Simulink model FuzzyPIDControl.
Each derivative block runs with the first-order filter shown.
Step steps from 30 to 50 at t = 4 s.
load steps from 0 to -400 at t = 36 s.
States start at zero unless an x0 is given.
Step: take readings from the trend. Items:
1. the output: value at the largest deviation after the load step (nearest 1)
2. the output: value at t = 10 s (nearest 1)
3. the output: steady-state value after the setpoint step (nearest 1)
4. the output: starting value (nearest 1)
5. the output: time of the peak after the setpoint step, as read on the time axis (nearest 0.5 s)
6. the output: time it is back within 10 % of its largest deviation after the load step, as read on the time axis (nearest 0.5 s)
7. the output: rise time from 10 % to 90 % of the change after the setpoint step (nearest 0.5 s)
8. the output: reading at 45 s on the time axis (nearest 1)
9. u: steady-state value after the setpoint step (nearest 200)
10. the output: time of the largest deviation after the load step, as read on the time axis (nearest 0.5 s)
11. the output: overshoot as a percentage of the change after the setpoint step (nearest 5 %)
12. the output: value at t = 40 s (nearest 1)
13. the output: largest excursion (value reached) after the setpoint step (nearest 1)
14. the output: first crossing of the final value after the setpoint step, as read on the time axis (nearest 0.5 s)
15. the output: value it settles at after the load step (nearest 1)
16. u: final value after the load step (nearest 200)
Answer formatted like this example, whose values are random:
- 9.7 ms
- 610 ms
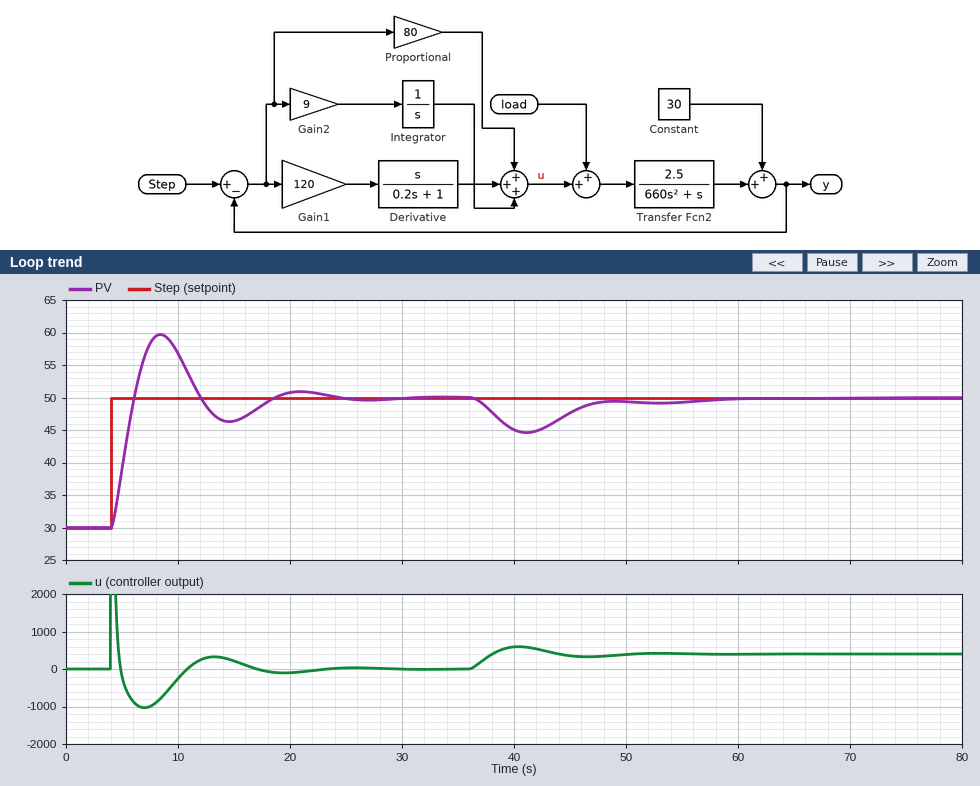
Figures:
- 45
- 57
- 50
- 30
- 8.5 s
- 56.5 s
- 1.5 s
- 48
- 0
- 41.0 s
- 50 %
- 45
- 60
- 6.0 s
- 50
- 400
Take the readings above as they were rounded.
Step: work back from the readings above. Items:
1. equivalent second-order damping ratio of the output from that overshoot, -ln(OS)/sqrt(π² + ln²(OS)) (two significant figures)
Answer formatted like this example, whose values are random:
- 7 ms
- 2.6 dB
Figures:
- 0.22
